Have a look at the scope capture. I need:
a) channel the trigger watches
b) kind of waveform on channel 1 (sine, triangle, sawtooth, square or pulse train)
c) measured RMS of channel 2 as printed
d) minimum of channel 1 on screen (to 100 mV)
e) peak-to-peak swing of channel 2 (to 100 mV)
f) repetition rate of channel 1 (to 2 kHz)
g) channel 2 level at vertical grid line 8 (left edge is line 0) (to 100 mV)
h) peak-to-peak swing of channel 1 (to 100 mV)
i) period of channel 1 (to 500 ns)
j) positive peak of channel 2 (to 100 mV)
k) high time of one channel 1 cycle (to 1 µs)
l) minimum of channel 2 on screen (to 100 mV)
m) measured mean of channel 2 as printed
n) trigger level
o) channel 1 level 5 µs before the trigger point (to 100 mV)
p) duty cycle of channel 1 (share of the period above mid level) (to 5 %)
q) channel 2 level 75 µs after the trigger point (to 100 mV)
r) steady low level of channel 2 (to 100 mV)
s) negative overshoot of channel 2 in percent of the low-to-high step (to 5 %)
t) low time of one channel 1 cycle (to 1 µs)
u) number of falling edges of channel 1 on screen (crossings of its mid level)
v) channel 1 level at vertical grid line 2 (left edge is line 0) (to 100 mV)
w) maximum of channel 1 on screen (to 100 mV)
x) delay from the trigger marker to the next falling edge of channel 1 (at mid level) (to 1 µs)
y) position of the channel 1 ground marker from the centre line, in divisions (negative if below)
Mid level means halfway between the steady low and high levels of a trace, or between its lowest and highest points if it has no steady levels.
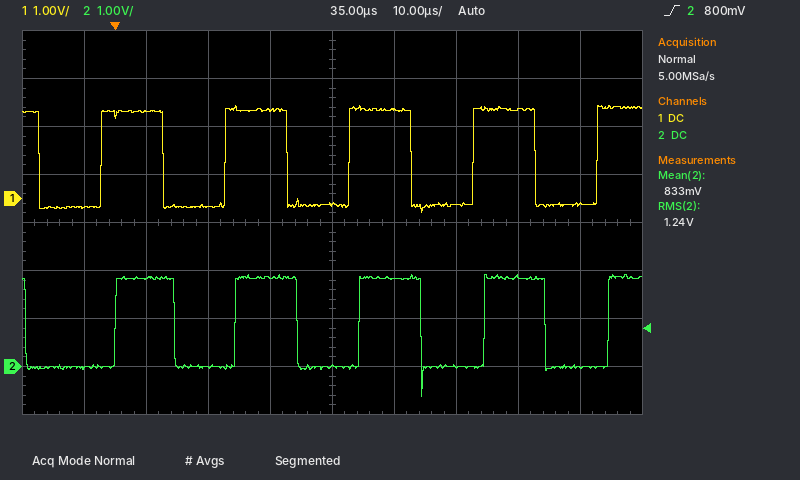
channel 2
square
1.24 V
-300 mV
2.5 V
50 kHz
1.9 V
2.2 V
20.0 µs
1.9 V
10 µs
-600 mV
833 mV
800 mV
-200 mV
50 %
0.0 V
0.0 V
35 %
10 µs
5
1.8 V
1.9 V
8 µs
+0.5 div
